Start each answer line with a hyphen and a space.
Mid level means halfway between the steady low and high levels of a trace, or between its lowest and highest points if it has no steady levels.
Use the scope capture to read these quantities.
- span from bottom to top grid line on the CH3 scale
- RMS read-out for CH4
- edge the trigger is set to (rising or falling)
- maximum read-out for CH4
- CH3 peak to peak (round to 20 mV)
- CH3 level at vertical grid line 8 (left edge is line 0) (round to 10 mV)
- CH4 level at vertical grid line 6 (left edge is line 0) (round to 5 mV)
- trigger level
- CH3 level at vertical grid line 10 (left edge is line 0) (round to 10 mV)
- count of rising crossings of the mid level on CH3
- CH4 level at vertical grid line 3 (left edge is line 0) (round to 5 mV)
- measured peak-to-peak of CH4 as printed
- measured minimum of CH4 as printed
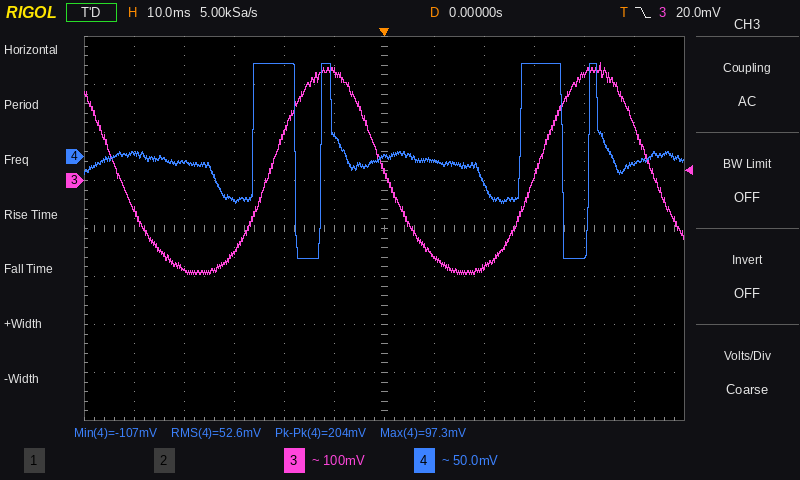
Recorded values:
- 800 mV
- 52.6 mV
- falling
- 97.3 mV
- 440 mV
- -180 mV
- 0 mV
- 20.0 mV
- 220 mV
- 2
- -45 mV
- 204 mV
- -107 mV
